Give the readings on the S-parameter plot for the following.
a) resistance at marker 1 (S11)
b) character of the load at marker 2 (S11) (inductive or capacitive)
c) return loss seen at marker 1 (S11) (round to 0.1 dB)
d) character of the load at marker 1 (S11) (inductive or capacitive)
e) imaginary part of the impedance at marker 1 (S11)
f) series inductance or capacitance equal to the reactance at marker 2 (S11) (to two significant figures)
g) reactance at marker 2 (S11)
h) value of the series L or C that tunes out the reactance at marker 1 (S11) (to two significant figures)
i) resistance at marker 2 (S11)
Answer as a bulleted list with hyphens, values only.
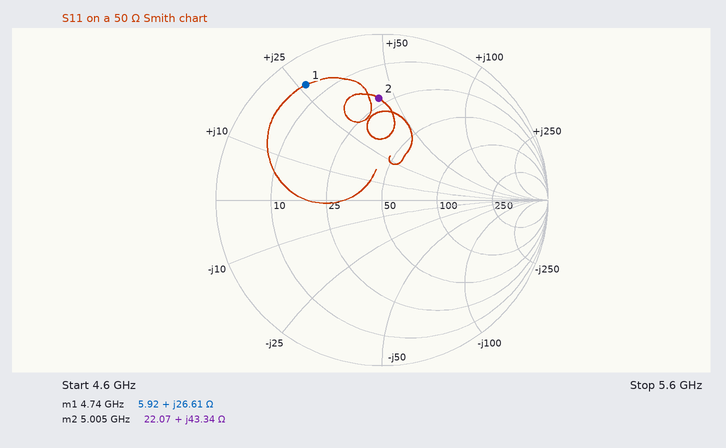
- 5.92 Ω
- inductive
- 1.6 dB
- inductive
- +26.61 Ω
- 1.4 nH
- +43.34 Ω
- 1.3 pF
- 22.07 Ω
